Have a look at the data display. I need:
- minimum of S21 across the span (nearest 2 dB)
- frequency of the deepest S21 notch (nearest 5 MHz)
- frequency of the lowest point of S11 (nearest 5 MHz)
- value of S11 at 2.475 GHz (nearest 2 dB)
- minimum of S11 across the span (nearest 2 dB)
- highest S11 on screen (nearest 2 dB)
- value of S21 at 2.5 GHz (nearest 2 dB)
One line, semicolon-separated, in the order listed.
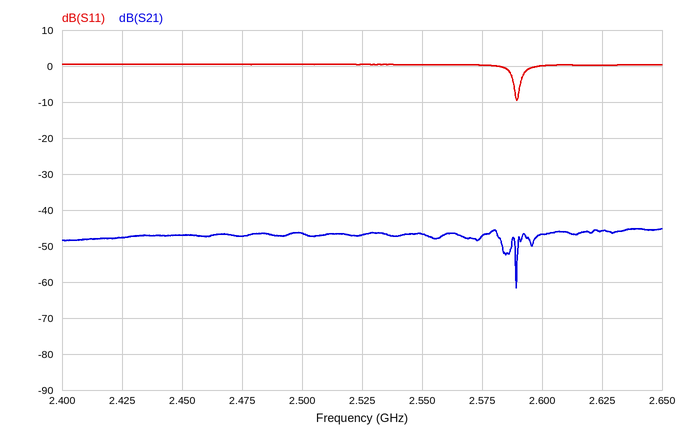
-62 dB; 2.590 GHz; 2.590 GHz; 0 dB; -10 dB; 0 dB; -46 dB
